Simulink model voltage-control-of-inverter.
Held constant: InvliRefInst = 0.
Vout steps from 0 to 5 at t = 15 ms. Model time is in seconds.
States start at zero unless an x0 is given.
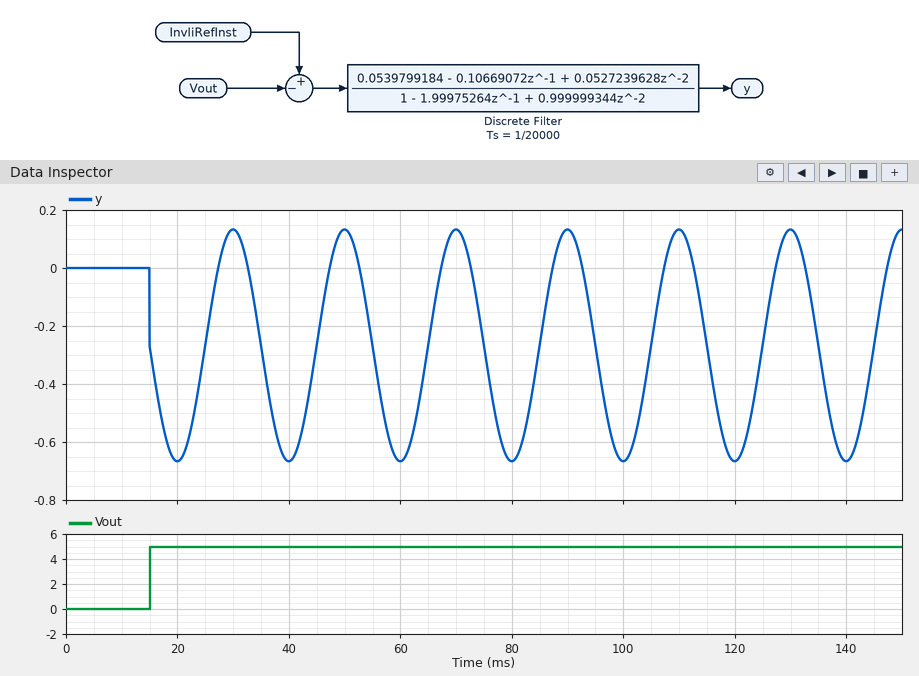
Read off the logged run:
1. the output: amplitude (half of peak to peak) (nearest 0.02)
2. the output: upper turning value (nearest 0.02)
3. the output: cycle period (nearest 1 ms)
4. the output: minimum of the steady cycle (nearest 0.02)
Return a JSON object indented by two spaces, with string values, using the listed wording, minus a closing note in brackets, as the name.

{
  "the output: amplitude (half of peak to peak)": "0.40",
  "the output: upper turning value": "0.14",
  "the output: cycle period": "20 ms",
  "the output: minimum of the steady cycle": "-0.66"
}
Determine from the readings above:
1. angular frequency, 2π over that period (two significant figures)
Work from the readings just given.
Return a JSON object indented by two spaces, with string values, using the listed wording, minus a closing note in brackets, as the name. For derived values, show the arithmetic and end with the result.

{
  "angular frequency, 2π over that period": "2π / 20 = 0.31 rad/ms"
}
